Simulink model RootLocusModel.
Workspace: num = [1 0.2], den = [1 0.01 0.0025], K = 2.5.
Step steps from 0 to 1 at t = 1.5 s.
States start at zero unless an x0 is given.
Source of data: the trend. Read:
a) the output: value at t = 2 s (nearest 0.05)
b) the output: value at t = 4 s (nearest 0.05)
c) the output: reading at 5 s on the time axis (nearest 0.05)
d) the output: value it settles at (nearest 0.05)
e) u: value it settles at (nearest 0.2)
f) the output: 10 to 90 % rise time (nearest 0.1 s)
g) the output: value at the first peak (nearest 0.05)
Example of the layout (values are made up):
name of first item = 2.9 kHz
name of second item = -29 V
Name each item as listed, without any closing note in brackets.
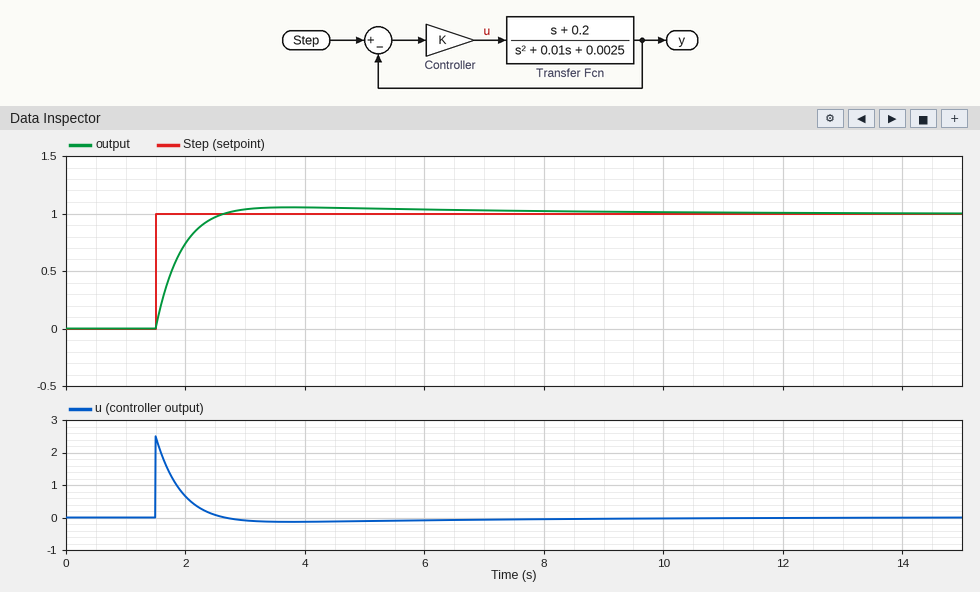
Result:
the output: value at t = 2 s = 0.75
the output: value at t = 4 s = 1.05
the output: reading at 5 s on the time axis = 1.05
the output: value it settles at = 1.00
u: value it settles at = 0.0
the output: 10 to 90 % rise time = 0.7 s
the output: value at the first peak = 1.05
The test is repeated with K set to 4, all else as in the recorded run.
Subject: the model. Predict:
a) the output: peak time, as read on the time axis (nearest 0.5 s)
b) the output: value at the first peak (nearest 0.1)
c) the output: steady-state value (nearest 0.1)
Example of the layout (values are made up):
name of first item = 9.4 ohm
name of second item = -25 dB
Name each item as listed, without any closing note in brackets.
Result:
the output: peak time, as read on the time axis = 3.0 s
the output: value at the first peak = 1.0
the output: steady-state value = 1.0
